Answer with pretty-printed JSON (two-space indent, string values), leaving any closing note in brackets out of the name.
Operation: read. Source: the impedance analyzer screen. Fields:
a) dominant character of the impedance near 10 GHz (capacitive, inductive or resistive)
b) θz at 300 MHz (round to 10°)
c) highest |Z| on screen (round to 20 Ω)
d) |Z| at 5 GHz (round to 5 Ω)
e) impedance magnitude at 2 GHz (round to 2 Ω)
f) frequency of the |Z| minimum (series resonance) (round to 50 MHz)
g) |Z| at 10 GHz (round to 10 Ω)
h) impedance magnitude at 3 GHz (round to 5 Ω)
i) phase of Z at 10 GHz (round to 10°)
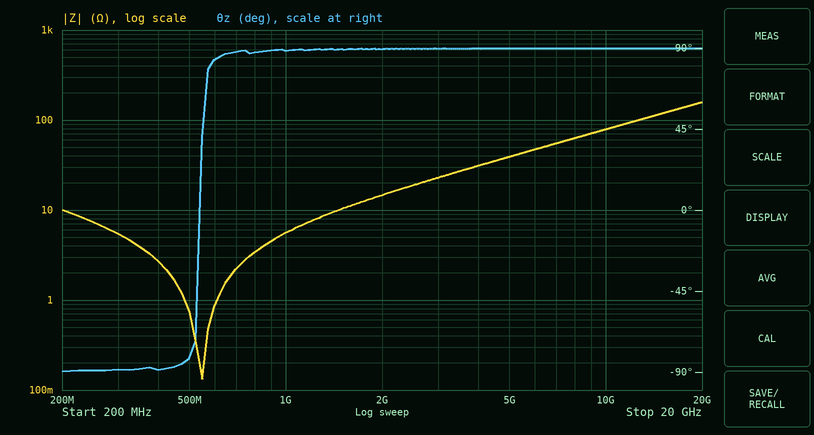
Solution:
{
  "dominant character of the impedance near 10 GHz": "inductive",
  "θz at 300 MHz": "-90°",
  "highest |Z| on screen": "160 Ω",
  "|Z| at 5 GHz": "40 Ω",
  "impedance magnitude at 2 GHz": "14 Ω",
  "frequency of the |Z| minimum (series resonance)": "550 MHz",
  "|Z| at 10 GHz": "80 Ω",
  "impedance magnitude at 3 GHz": "25 Ω",
  "phase of Z at 10 GHz": "90°"
}
